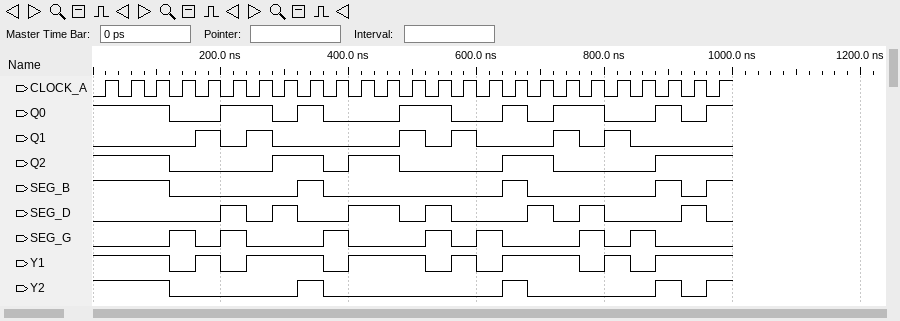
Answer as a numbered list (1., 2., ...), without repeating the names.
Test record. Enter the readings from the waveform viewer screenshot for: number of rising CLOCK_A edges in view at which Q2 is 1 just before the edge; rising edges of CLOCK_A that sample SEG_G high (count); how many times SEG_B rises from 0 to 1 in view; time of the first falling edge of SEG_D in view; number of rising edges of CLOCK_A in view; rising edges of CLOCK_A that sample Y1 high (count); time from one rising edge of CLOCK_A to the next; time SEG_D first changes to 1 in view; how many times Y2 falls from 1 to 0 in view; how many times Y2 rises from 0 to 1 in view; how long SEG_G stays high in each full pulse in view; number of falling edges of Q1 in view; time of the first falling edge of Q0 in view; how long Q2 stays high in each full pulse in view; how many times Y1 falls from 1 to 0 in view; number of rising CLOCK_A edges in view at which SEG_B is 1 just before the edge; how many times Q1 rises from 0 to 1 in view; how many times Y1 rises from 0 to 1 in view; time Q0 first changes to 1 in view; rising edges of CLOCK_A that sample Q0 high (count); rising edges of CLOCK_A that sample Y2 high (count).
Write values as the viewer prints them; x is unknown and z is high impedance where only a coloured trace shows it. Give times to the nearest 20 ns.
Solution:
1. 12
2. 7
3. 4
4. 240 ns
5. 25
6. 18
7. 40 ns
8. 200 ns
9. 4
10. 4
11. 40 ns, 40 ns, 40 ns, 40 ns, 40 ns, 40 ns, 40 ns
12. 6
13. 120 ns
14. 80 ns, 80 ns, 80 ns
15. 7
16. 7
17. 6
18. 7
19. 200 ns
20. 13
21. 7
